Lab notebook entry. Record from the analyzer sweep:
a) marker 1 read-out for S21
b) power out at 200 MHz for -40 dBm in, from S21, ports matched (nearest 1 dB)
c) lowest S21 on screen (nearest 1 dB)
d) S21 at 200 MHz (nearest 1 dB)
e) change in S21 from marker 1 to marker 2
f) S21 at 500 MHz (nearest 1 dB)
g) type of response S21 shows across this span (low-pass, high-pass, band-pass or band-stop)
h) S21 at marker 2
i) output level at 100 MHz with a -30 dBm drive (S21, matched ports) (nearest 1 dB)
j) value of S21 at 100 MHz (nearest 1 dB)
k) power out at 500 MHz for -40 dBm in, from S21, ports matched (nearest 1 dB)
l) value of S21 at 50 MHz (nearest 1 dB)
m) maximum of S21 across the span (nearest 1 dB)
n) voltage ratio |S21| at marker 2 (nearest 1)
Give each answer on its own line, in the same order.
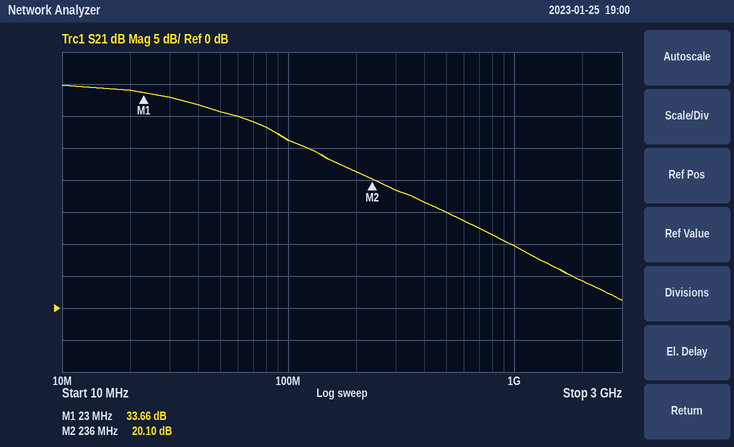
33.66 dB
-19 dBm
1 dB
21 dB
-13.56 dB
15 dB
low-pass
20.10 dB
-4 dBm
26 dB
-25 dBm
31 dB
35 dB
10
